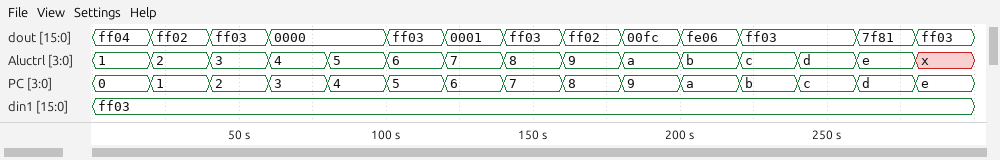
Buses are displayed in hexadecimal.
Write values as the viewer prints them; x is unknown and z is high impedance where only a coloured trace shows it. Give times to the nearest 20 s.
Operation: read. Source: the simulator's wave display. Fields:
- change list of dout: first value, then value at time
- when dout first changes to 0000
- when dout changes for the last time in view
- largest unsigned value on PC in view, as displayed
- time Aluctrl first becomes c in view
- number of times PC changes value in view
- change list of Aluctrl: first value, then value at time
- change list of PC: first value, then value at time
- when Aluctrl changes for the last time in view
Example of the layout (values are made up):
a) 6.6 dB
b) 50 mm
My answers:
a) ff04, ff02 at 20 s, ff03 at 40 s, 0000 at 60 s, ff03 at 100 s, 0001 at 120 s, ff03 at 140 s, ff02 at 160 s, 00fc at 180 s, fe06 at 200 s, ff03 at 220 s, 7f81 at 260 s, ff03 at 280 s
b) 60 s
c) 280 s
d) e
e) 220 s
f) 14
g) 1, 2 at 20 s, 3 at 40 s, 4 at 60 s, 5 at 80 s, 6 at 100 s, 7 at 120 s, 8 at 140 s, 9 at 160 s, a at 180 s, b at 200 s, c at 220 s, d at 240 s, e at 260 s, x at 280 s
h) 0, 1 at 20 s, 2 at 40 s, 3 at 60 s, 4 at 80 s, 5 at 100 s, 6 at 120 s, 7 at 140 s, 8 at 160 s, 9 at 180 s, a at 200 s, b at 220 s, c at 240 s, d at 260 s, e at 280 s
i) 280 s
